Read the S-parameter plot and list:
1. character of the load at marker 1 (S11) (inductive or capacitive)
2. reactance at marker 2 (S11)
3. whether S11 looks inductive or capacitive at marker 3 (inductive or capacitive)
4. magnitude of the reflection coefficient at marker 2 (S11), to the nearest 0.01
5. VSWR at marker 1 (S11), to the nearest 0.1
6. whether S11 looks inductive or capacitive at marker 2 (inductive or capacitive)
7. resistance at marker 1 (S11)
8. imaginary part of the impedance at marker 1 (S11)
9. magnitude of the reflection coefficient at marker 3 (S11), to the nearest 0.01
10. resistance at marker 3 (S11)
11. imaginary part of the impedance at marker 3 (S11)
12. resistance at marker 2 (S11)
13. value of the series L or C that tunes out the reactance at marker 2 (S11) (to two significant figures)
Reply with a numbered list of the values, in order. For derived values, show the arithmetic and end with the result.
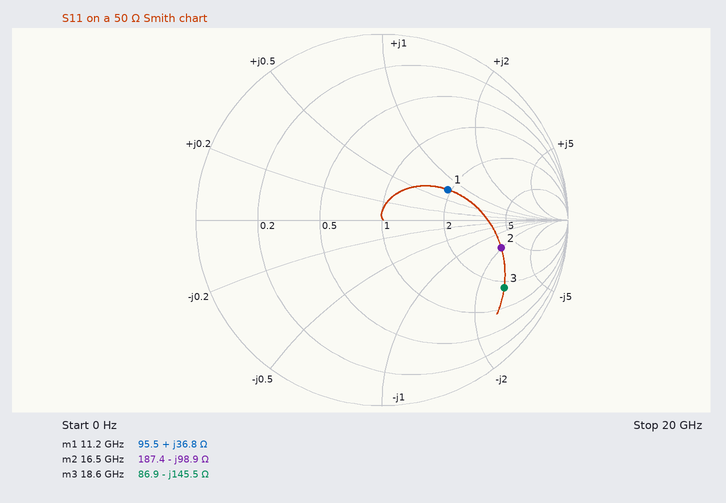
1. inductive
2. -98.9 Ω
3. capacitive
4. 0.66
5. 2.3
6. capacitive
7. 95.5 Ω
8. +36.8 Ω
9. 0.75
10. 86.9 Ω
11. -145.5 Ω
12. 187.4 Ω
13. L = 98.9 Ω/(2π × 16.5 GHz) ≈ 954 pH, so 950 pH to two significant figures
